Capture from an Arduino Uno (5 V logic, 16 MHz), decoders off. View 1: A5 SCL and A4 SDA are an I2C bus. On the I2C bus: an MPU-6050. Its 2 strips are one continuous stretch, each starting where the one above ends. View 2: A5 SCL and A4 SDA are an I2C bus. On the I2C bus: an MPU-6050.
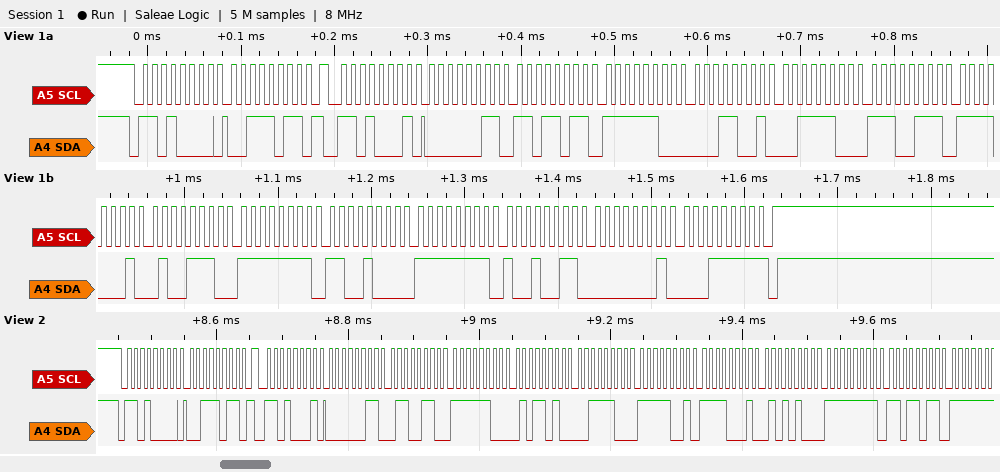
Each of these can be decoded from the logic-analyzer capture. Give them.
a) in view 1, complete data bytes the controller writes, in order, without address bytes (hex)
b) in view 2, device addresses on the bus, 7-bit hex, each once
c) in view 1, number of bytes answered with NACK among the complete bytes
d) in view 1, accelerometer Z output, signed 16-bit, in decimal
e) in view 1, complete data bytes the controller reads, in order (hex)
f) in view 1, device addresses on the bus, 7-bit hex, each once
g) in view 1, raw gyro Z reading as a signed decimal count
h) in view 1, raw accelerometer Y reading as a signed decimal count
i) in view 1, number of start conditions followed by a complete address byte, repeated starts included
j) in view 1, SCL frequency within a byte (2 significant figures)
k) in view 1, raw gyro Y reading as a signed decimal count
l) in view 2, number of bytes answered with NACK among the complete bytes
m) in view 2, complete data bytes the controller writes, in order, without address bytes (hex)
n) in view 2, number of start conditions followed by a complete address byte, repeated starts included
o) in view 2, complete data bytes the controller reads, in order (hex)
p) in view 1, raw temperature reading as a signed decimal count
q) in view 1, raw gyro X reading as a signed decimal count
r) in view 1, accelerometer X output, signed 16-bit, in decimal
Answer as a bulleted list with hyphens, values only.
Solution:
- 3B
- 0x68
- 1
- 15591
- 03 DB FC 19 3C E7 F1 4E FF C8 FF 93 01 1F
- 0x68
- 287
- -999
- 2
- 100 kHz
- -109
- 0
- 3B
- 2
- 03 66 FC 5A 3C F9 F1 54 FF DB
- -3762
- -56
- 987
